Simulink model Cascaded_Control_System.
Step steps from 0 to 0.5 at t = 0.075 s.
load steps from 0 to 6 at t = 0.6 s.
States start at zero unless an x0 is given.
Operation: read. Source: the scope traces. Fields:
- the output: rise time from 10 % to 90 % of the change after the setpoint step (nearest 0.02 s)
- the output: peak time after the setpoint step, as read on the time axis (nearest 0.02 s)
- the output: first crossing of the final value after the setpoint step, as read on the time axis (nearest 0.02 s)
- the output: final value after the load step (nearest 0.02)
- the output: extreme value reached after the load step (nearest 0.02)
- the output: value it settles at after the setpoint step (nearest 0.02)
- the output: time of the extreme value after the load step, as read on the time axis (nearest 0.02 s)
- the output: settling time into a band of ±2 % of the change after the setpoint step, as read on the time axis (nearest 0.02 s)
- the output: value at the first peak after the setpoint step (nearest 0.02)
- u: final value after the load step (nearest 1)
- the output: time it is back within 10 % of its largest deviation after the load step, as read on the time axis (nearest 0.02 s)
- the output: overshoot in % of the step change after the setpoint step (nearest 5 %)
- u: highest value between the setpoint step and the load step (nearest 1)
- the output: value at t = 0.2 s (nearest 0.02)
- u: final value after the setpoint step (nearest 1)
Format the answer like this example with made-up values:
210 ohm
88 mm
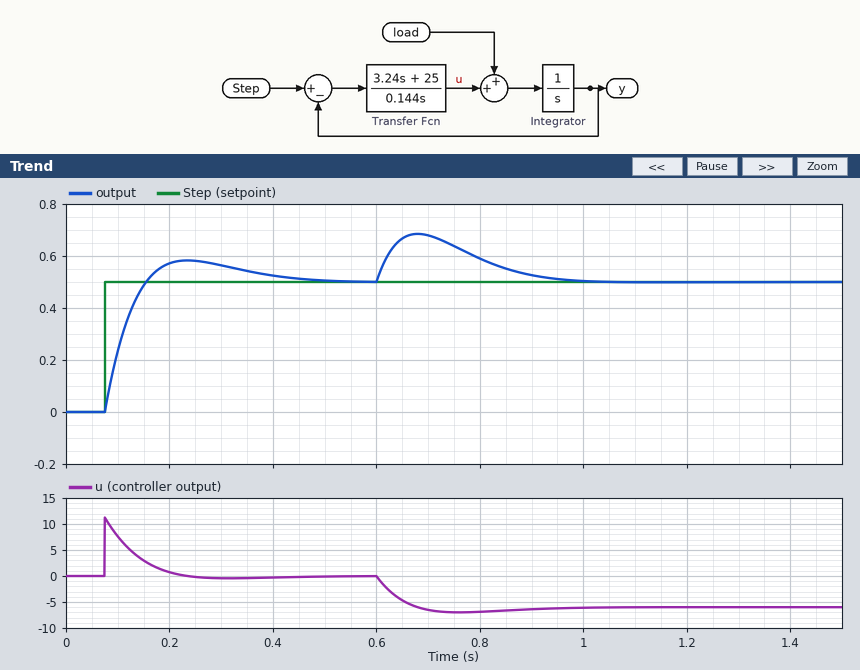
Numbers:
0.06 s
0.24 s
0.16 s
0.50
0.68
0.50
0.68 s
0.46 s
0.58
-6
0.92 s
15 %
11
0.58
0
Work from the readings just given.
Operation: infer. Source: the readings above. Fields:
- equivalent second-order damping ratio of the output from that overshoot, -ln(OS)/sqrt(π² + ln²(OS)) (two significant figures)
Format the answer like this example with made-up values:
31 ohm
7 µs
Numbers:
0.52
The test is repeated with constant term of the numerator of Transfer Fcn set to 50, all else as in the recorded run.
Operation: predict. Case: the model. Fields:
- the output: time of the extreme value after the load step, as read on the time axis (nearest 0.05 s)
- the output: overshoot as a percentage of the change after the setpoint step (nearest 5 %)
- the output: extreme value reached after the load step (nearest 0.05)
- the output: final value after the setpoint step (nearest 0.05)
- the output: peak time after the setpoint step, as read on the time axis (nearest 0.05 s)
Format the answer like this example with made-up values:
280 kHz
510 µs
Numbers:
0.65 s
25 %
0.65
0.50
0.20 s
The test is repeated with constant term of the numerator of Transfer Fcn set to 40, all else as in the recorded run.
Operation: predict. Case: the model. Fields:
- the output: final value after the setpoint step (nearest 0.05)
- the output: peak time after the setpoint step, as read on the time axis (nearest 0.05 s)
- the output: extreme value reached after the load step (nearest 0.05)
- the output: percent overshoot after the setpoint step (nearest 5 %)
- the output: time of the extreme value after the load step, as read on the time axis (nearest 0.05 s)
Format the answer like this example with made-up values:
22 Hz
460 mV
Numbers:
0.50
0.20 s
0.65
20 %
0.65 s
